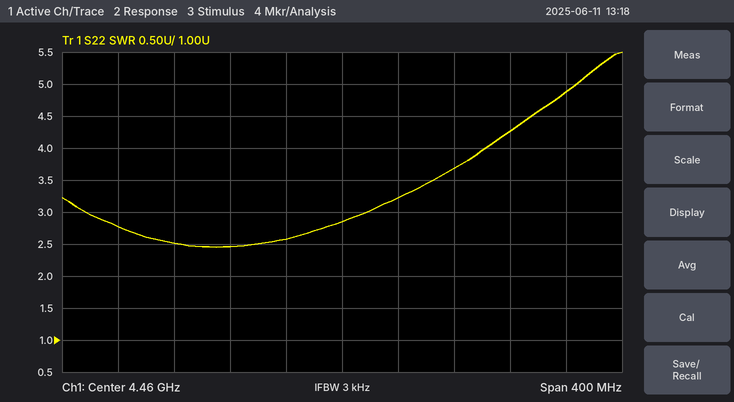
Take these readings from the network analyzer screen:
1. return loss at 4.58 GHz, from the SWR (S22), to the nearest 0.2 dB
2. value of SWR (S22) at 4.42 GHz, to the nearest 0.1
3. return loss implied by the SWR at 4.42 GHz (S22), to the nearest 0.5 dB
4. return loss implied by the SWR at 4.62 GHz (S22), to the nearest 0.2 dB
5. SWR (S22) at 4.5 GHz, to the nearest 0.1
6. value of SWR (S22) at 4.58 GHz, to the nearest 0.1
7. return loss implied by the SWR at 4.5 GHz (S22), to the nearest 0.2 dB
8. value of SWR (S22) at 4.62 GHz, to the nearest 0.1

4.2 dB
2.6
7.0 dB
3.6 dB
3.2
4.3
5.6 dB
4.9
